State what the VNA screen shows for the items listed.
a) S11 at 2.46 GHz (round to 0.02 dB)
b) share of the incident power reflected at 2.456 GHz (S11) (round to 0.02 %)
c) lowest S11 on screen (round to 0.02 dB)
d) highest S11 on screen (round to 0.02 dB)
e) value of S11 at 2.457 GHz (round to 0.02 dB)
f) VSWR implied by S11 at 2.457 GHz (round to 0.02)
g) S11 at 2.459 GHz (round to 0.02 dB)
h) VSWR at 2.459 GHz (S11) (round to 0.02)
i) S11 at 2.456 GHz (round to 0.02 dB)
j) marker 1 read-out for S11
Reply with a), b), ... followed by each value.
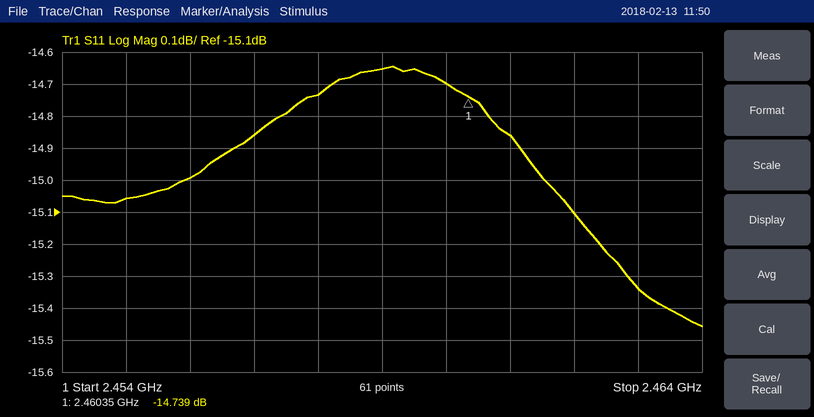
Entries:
a) -14.70 dB
b) 3.16 %
c) -15.46 dB
d) -14.64 dB
e) -14.86 dB
f) 1.44
g) -14.66 dB
h) 1.46
i) -15.00 dB
j) -14.739 dB
